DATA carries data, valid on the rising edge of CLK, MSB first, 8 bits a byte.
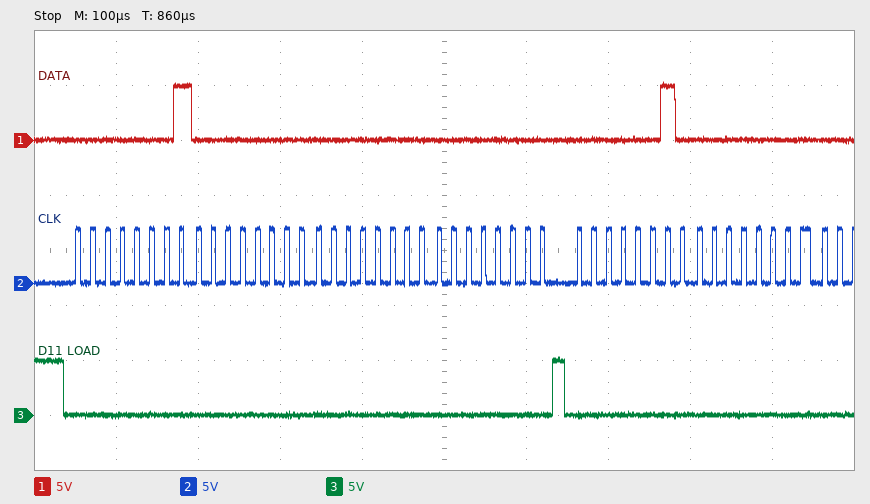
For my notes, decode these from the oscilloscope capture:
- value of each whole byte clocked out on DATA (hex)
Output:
0x01 0x00 0x00 0x00 0x02 0x00
